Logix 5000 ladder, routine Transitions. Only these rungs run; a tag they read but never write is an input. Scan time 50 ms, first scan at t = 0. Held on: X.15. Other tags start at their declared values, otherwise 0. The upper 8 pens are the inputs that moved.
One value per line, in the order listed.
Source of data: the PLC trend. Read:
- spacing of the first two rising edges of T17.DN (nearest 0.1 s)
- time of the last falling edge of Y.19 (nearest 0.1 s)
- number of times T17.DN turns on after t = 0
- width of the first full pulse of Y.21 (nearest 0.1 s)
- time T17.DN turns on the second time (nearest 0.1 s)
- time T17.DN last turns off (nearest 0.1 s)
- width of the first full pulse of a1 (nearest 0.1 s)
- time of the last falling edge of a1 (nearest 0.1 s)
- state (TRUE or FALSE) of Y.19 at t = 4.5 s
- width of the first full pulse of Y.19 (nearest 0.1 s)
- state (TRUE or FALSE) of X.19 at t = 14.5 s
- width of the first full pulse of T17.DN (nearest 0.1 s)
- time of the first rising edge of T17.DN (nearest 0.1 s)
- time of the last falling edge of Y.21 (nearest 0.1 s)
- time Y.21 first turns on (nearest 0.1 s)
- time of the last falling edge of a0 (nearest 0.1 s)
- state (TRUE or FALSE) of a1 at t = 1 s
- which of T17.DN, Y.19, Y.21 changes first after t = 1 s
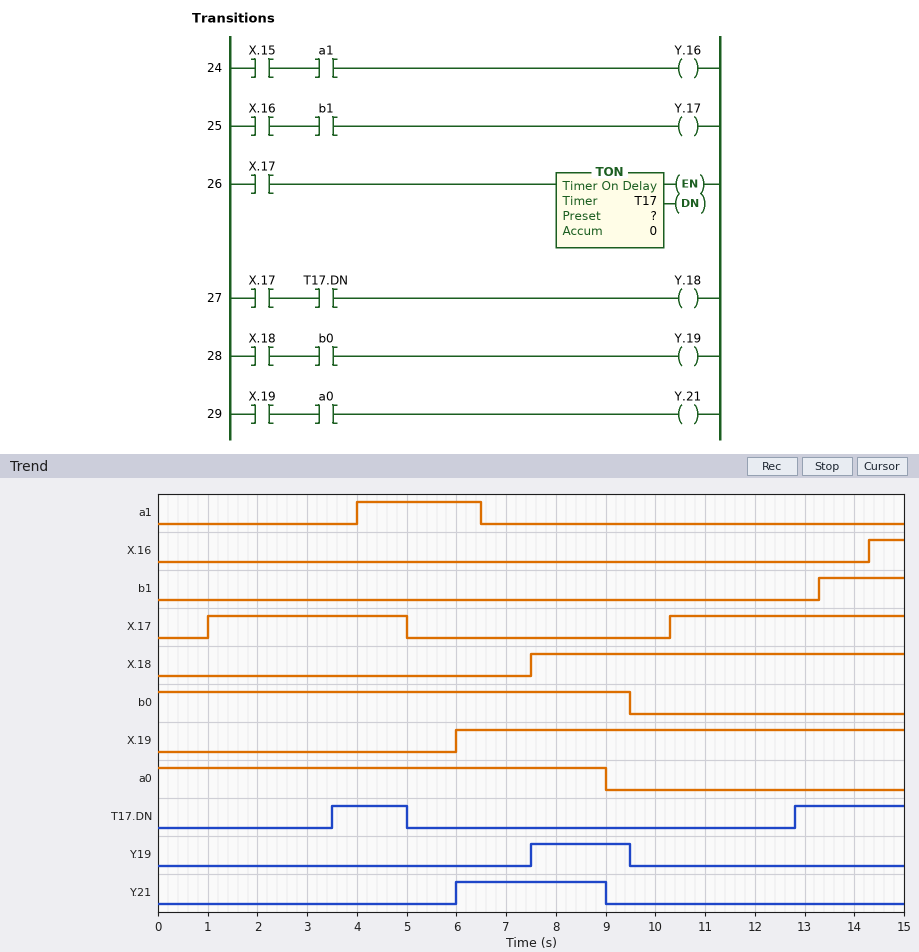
9.3 s
9.5 s
2
3.0 s
12.8 s
5.0 s
2.5 s
6.5 s
FALSE
2.0 s
TRUE
1.5 s
3.5 s
9.0 s
6.0 s
9.0 s
FALSE
T17.DN
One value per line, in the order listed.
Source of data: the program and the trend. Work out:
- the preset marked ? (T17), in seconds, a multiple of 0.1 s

2.5 s
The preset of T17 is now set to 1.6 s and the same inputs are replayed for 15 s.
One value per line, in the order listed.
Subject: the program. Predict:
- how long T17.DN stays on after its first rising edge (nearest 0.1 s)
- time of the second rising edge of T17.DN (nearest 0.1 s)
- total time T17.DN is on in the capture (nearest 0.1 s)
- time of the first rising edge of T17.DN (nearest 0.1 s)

2.4 s
11.9 s
5.5 s
2.6 s
